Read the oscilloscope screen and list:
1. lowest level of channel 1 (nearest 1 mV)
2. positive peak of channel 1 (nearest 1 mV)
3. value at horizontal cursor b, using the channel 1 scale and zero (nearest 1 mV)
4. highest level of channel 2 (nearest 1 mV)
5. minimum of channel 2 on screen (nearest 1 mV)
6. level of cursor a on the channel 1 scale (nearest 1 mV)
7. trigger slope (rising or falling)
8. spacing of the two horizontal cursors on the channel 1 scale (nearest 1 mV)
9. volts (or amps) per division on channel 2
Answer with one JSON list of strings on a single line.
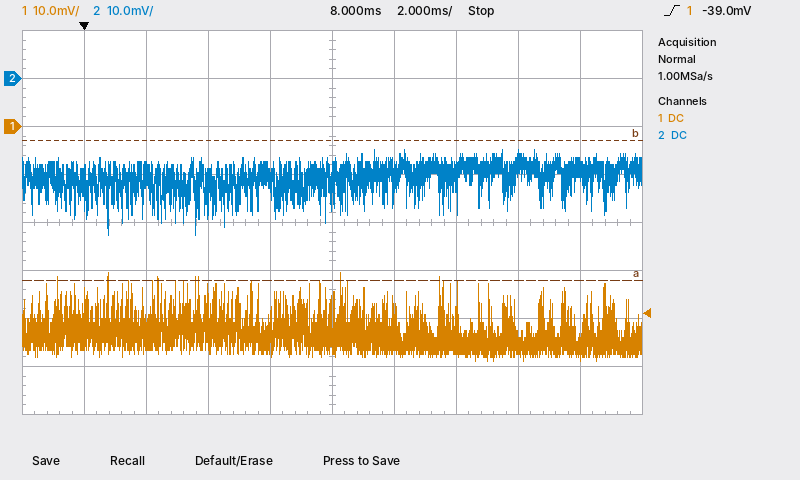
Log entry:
["-49 mV", "-30 mV", "-3 mV", "-15 mV", "-32 mV", "-32 mV", "rising", "29 mV", "10 mV"]
